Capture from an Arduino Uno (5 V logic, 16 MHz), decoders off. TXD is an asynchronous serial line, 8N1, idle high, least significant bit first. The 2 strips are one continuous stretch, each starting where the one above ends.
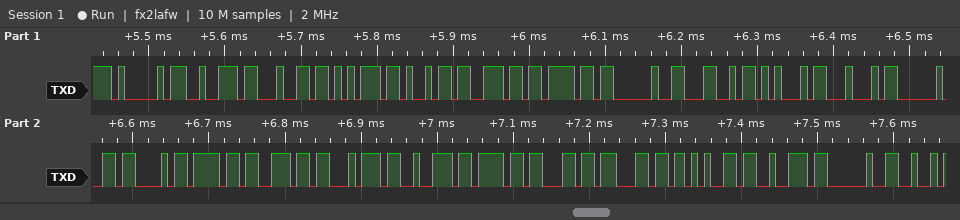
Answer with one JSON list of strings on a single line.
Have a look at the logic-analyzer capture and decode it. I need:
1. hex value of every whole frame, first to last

["0x41 0x72 0x64 0x75 0x69 0x6E 0x6F 0x20 0x4C 0x45 0x44 0x20 0x43 0x6F 0x6E 0x74 0x72 0x6F 0x6C 0x6C 0x65 0x72 0x20"]
